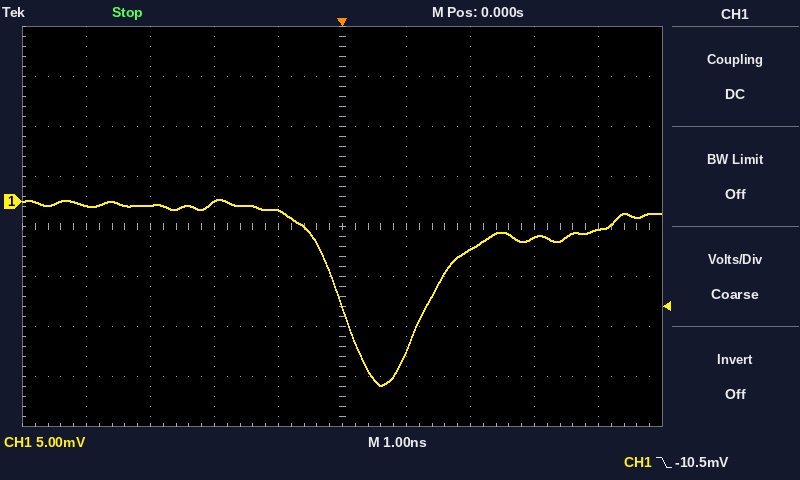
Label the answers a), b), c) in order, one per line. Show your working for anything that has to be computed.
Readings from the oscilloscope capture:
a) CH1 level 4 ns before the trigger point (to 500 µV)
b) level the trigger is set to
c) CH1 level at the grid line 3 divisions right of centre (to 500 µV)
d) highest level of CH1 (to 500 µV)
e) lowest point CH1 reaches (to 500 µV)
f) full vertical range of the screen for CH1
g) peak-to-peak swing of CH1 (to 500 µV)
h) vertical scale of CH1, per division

a) -500 µV
b) -10.5 mV
c) -3.5 mV
d) 0.0 mV
e) -18.5 mV
f) 40 mV
g) 0.0 mV − (-18.5 mV) = 18.5 mV
h) 5 mV
